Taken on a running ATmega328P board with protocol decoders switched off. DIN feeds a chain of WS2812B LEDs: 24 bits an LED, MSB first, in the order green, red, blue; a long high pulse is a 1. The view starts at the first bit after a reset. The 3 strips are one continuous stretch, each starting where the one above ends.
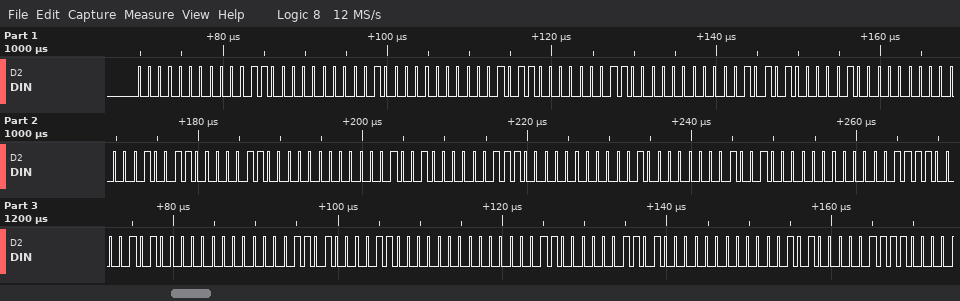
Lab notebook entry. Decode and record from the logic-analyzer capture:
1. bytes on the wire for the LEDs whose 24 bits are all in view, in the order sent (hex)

00 18 01 00 16 03 00 15 04 00 13 06 00 12 07 00 10 09 00 0F 0A 00 0D 0C 00 0C 0D 00 0A 0F
